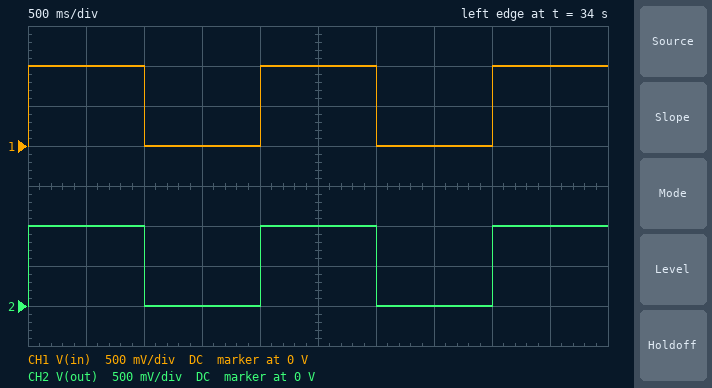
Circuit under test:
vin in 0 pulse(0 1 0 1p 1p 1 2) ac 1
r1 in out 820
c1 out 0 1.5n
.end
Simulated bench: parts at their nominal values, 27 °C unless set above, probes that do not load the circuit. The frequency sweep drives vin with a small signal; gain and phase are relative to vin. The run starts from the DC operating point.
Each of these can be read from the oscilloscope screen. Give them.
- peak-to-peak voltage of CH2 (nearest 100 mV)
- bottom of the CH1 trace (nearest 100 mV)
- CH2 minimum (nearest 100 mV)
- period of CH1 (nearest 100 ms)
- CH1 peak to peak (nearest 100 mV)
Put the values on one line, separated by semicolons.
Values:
1.0 V; 0 V; 0 V; 2.0 s; 1.0 V
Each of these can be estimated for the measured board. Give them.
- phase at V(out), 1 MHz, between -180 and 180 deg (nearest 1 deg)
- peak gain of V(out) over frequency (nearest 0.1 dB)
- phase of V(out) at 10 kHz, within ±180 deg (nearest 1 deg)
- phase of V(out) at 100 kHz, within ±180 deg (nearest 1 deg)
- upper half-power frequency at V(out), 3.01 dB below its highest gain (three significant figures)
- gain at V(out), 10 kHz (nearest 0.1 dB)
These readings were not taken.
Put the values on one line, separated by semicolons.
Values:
-83 deg; 0 dB; -4 deg; -38 deg; 129 kHz; 0 dB
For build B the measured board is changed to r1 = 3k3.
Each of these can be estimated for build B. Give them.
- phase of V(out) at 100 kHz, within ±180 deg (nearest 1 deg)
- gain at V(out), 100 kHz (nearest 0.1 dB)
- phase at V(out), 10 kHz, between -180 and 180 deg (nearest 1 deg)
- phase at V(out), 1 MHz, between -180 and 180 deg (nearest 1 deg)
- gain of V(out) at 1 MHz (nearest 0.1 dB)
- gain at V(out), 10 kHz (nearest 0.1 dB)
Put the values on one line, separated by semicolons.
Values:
-72 deg; -10.3 dB; -17 deg; -88 deg; -29.9 dB; -0.4 dB
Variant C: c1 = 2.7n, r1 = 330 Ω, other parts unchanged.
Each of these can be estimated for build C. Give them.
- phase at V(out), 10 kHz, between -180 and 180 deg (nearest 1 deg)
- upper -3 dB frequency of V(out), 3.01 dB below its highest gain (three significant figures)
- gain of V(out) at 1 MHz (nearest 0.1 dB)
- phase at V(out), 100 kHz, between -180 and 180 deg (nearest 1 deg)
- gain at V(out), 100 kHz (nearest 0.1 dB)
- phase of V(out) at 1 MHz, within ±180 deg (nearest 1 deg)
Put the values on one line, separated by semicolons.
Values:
-3 deg; 179 kHz; -15.1 dB; -29 deg; -1.2 dB; -80 deg
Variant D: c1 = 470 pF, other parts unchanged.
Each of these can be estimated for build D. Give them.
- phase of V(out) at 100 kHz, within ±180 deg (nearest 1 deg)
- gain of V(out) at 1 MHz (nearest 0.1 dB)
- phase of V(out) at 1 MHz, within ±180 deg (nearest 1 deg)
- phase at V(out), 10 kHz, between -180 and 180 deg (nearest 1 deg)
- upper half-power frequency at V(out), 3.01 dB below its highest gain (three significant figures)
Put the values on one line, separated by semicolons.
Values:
-14 deg; -8.4 dB; -68 deg; -1 deg; 413 kHz
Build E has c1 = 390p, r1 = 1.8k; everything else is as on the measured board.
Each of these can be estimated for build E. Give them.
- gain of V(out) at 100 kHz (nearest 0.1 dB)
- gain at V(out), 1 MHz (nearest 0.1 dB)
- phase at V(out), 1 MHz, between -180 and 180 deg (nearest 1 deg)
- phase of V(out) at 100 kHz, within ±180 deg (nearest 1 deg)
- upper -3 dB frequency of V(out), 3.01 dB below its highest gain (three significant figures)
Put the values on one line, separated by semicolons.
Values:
-0.8 dB; -13.1 dB; -77 deg; -24 deg; 227 kHz
